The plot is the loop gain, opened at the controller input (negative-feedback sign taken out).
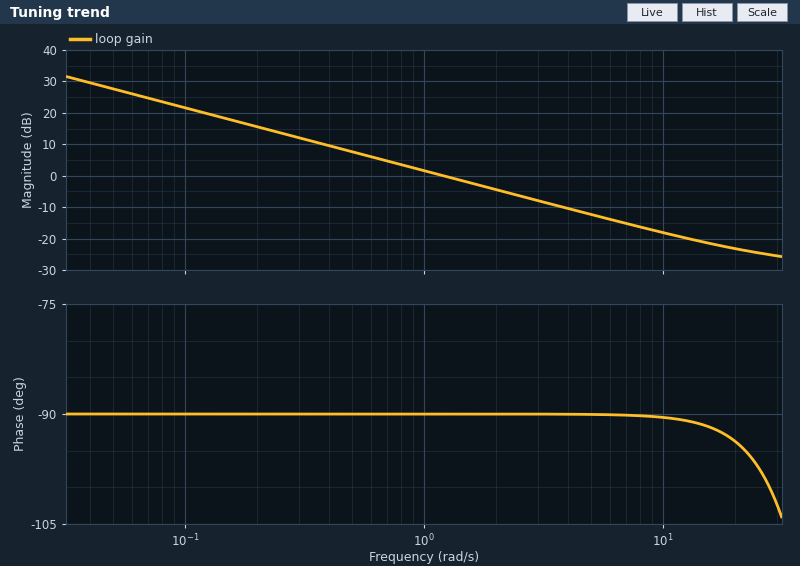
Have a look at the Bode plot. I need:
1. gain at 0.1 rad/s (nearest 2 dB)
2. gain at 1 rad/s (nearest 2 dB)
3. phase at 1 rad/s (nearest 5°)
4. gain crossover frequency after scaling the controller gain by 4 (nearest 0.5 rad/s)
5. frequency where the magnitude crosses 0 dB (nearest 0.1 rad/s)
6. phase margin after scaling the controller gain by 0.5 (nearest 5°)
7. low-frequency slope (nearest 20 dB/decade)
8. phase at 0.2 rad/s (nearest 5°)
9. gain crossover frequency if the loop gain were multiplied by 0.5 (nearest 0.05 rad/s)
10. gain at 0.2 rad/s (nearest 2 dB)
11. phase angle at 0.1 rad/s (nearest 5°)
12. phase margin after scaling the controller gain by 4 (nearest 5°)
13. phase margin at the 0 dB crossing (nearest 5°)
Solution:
22 dB
2 dB
-90°
5.0 rad/s
1.2 rad/s
90°
-20 dB/decade
-90°
0.60 rad/s
16 dB
-90°
90°
90°
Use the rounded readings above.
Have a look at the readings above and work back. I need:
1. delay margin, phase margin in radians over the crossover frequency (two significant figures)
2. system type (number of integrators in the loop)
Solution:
1.3 s
1
